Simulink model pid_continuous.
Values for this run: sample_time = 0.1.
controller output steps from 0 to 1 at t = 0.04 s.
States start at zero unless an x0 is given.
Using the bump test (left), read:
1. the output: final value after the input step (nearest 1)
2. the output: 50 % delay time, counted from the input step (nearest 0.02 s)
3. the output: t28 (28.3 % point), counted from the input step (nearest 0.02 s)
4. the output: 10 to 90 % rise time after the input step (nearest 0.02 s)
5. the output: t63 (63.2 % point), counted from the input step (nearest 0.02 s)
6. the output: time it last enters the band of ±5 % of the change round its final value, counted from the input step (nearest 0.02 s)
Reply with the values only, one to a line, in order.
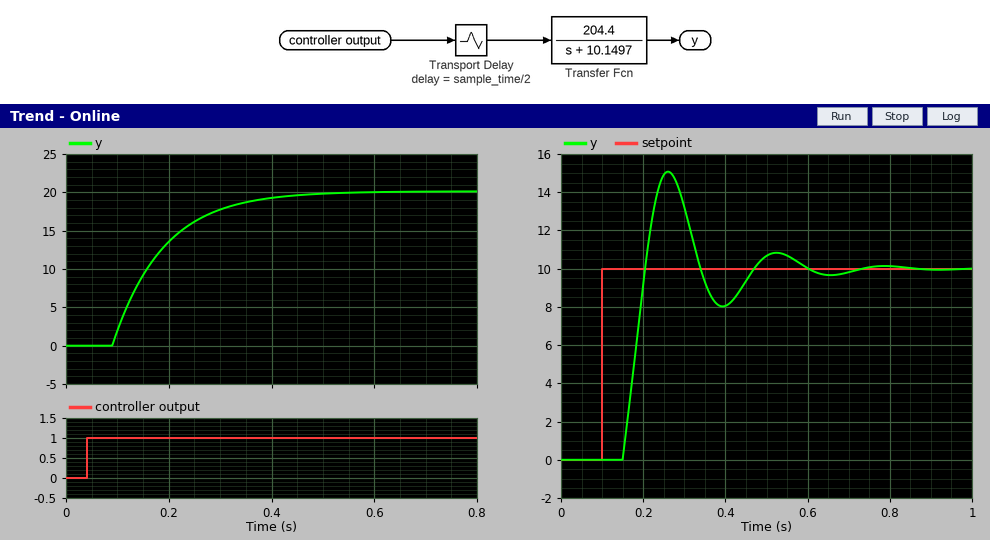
20
0.12 s
0.08 s
0.22 s
0.14 s
0.34 s
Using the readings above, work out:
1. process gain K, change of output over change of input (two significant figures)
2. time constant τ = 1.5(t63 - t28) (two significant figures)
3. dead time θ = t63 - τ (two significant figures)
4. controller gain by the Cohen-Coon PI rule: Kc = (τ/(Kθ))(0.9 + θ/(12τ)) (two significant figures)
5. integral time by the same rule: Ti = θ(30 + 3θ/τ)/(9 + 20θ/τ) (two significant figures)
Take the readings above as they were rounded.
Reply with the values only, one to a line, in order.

20
0.090 s
0.050 s
0.085
0.079 s
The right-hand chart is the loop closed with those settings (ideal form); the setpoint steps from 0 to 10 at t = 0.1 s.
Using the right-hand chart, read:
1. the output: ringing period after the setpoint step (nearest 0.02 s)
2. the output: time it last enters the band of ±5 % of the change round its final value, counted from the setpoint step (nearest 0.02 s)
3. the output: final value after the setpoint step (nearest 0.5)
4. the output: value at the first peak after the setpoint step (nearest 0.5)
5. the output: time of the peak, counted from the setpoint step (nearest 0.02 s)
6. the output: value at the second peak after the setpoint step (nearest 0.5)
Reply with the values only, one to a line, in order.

0.26 s
0.46 s
10.0
15.0
0.16 s
11.0
